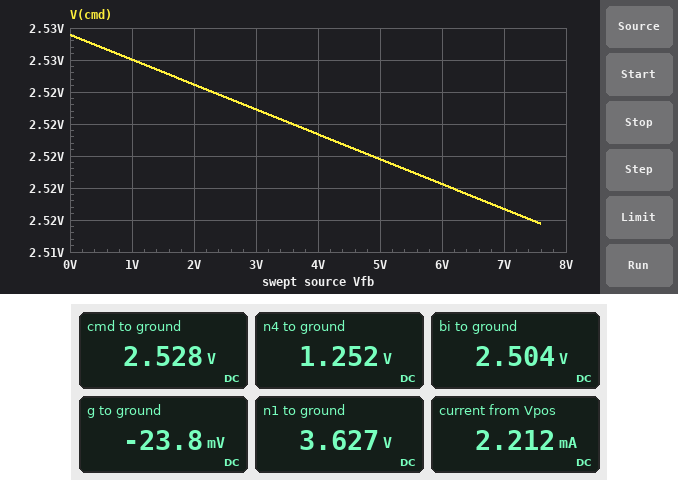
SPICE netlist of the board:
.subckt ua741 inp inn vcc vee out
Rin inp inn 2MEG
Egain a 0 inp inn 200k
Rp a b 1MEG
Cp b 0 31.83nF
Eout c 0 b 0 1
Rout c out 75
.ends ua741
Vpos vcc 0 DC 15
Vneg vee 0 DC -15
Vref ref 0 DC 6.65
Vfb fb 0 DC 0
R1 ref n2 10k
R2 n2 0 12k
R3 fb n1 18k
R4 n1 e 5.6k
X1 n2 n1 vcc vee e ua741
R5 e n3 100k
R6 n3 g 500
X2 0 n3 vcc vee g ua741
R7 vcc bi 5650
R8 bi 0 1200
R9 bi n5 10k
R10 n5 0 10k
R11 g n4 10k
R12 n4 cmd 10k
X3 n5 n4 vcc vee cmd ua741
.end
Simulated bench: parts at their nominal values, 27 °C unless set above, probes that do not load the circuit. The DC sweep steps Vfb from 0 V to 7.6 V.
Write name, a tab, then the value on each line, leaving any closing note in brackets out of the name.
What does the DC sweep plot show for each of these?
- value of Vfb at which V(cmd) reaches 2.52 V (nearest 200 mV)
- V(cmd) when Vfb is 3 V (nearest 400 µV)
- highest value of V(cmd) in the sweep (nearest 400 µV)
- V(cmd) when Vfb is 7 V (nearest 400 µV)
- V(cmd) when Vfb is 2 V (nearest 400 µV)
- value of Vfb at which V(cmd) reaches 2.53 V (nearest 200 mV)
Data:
value of Vfb at which V(cmd) reaches 2.52 V	6.2 V
V(cmd) when Vfb is 3 V	2.5228 V
highest value of V(cmd) in the sweep	2.5276 V
V(cmd) when Vfb is 7 V	2.5168 V
V(cmd) when Vfb is 2 V	2.5244 V
value of Vfb at which V(cmd) reaches 2.53 V	1.0 V
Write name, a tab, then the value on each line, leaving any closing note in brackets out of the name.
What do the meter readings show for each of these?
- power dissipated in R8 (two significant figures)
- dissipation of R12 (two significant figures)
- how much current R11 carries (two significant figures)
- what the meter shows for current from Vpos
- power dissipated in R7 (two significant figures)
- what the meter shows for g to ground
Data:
power dissipated in R8	5.2 mW
dissipation of R12	160 µW
how much current R11 carries	130 µA
what the meter shows for current from Vpos	2.212 mA
power dissipated in R7	28 mW
what the meter shows for g to ground	-23.8 mV
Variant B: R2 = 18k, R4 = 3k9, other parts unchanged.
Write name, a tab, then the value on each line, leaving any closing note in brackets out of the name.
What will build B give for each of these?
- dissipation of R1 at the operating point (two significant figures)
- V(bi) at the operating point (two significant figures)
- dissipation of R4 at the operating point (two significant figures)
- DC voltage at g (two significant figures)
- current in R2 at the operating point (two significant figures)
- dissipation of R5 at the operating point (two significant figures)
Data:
dissipation of R1 at the operating point	560 µW
V(bi) at the operating point	2.5 V
dissipation of R4 at the operating point	220 µW
DC voltage at g	-26 mV
current in R2 at the operating point	240 µA
dissipation of R5 at the operating point	270 µW
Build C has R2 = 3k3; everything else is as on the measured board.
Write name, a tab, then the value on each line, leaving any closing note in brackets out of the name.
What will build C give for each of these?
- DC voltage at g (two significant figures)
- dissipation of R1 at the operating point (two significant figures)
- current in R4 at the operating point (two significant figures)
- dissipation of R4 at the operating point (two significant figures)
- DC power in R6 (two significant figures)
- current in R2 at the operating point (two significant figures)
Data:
DC voltage at g	-11 mV
dissipation of R1 at the operating point	2.5 mW
current in R4 at the operating point	92 µA
dissipation of R4 at the operating point	47 µW
DC power in R6	230 nW
current in R2 at the operating point	500 µA
